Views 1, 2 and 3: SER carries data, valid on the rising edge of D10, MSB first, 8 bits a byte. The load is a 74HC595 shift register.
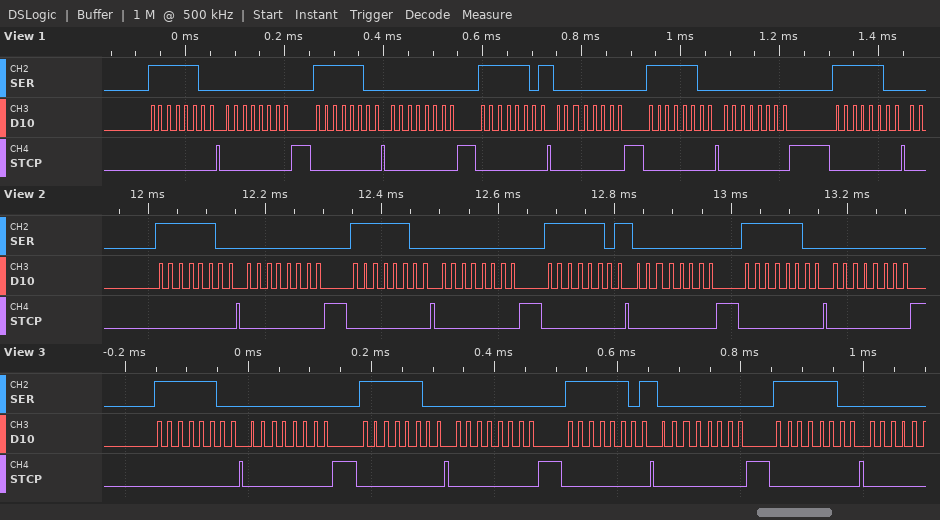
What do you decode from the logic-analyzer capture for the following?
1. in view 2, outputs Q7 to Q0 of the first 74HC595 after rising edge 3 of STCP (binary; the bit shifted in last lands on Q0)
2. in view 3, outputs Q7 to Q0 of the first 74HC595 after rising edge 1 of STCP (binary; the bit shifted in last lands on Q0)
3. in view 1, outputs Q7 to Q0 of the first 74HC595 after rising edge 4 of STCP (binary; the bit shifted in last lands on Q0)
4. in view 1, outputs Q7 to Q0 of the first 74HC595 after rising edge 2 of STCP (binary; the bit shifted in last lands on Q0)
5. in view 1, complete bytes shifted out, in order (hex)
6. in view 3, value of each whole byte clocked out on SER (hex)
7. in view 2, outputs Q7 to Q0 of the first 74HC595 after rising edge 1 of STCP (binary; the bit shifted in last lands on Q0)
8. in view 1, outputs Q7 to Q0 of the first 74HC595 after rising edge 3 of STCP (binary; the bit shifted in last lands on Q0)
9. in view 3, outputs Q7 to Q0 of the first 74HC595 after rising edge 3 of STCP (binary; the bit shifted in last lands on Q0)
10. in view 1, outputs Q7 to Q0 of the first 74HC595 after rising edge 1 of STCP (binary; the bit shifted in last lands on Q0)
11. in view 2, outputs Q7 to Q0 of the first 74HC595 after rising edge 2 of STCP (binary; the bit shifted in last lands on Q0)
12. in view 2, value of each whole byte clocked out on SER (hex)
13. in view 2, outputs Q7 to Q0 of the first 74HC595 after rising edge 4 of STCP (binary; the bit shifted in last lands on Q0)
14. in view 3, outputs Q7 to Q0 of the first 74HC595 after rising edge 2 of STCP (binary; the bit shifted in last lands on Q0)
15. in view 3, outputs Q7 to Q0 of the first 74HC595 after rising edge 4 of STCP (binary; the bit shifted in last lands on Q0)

11111100
11111100
00000000
00000000
FC 00 FC 00 FD 00 FC 00 FC
0xFC 0x00 0xFC 0x00 0xFD 0x00 0xFC
11111100
11111100
11111100
11111100
00000000
FC 00 FC 00 FD 00 FC 00
00000000
00000000
00000000
